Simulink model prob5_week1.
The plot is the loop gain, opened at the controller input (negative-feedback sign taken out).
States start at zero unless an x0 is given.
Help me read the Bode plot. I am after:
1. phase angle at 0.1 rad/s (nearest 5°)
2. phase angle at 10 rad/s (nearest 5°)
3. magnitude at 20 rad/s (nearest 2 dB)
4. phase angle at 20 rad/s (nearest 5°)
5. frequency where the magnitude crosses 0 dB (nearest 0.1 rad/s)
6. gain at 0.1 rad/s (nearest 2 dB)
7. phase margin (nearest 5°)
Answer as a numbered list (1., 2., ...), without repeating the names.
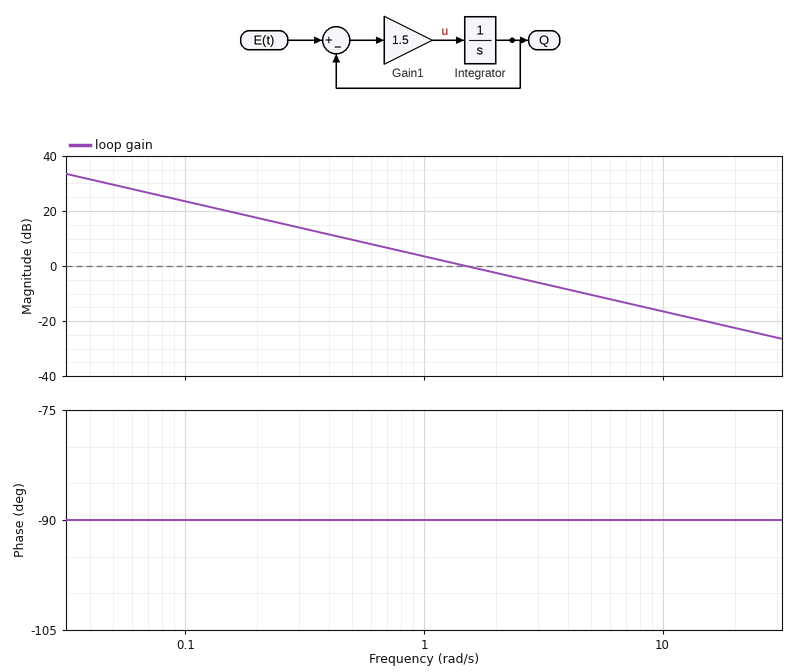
1. -90°
2. -90°
3. -22 dB
4. -90°
5. 1.5 rad/s
6. 24 dB
7. 90°
